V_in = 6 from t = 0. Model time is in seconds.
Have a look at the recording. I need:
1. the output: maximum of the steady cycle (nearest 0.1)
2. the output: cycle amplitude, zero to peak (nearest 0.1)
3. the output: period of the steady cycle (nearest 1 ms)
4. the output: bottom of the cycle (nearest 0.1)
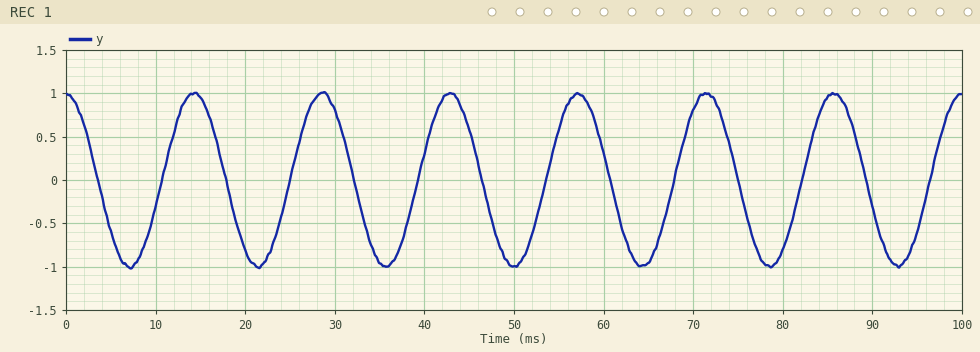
1.0
1.0
14 ms
-1.0
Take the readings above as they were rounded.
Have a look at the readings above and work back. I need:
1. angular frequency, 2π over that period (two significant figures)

0.45 rad/ms
